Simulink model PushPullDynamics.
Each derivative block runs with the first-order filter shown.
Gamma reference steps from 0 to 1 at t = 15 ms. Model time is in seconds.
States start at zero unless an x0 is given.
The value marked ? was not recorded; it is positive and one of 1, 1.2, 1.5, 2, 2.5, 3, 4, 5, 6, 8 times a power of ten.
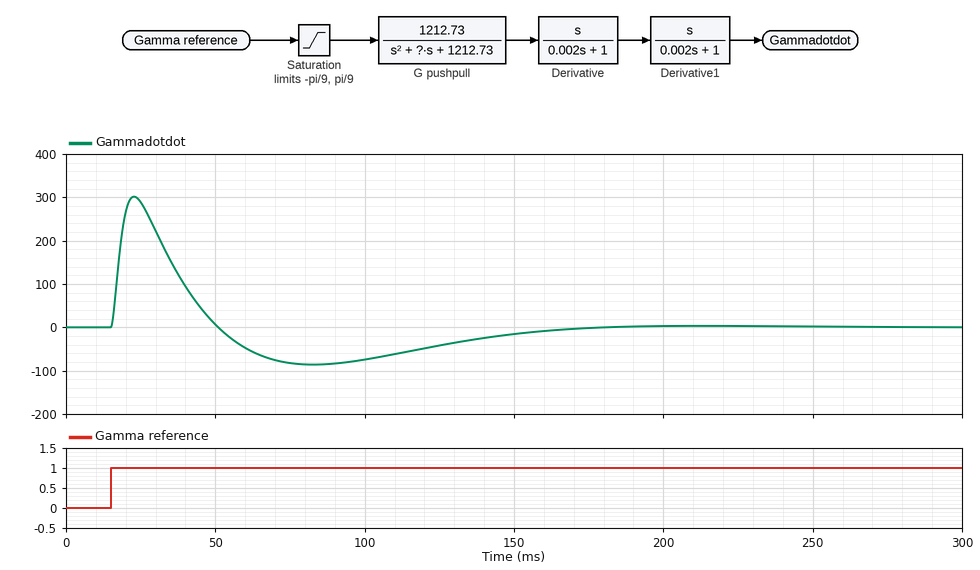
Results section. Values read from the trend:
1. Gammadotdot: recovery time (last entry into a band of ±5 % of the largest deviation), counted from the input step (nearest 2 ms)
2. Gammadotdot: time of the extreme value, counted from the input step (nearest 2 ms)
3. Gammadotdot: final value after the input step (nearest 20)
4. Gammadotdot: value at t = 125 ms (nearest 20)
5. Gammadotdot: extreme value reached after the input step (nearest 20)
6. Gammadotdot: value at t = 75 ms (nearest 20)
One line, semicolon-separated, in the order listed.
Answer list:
136 ms; 8 ms; 0; -40; 300; -80
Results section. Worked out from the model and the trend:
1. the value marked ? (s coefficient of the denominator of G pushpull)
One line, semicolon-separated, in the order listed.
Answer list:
50
